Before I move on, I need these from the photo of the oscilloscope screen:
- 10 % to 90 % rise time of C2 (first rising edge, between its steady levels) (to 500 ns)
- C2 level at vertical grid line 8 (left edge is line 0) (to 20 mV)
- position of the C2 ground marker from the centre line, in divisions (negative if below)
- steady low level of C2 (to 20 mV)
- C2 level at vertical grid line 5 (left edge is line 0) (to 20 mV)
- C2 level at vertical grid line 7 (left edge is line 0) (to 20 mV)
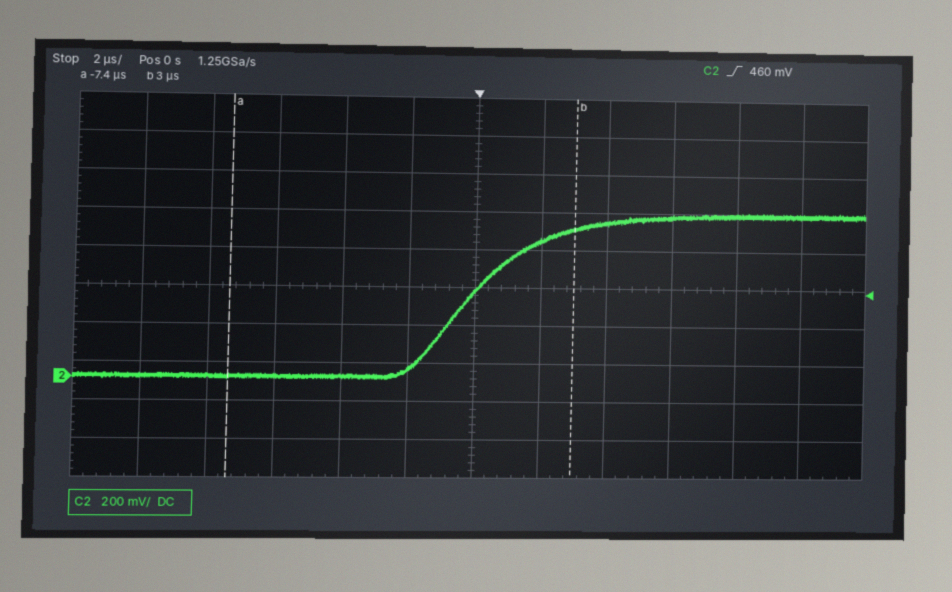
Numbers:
4.5 µs
820 mV
-2.4 div
0 mV
40 mV
720 mV
